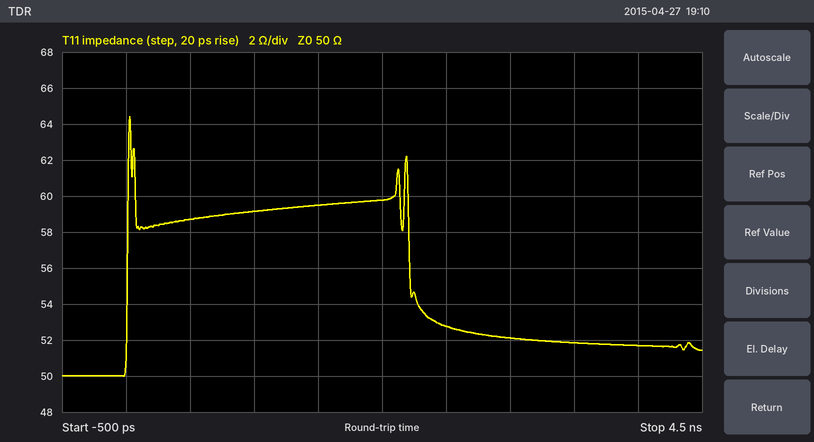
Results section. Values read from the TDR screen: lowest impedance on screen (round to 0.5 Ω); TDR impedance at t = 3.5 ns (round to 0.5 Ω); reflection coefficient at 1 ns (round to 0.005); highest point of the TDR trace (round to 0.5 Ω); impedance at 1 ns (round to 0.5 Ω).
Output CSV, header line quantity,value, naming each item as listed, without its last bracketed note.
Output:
quantity,value
lowest impedance on screen,50.0 Ω
TDR impedance at t = 3.5 ns,52.0 Ω
reflection coefficient at 1 ns,+0.085
highest point of the TDR trace,64.5 Ω
impedance at 1 ns,59.0 Ω
